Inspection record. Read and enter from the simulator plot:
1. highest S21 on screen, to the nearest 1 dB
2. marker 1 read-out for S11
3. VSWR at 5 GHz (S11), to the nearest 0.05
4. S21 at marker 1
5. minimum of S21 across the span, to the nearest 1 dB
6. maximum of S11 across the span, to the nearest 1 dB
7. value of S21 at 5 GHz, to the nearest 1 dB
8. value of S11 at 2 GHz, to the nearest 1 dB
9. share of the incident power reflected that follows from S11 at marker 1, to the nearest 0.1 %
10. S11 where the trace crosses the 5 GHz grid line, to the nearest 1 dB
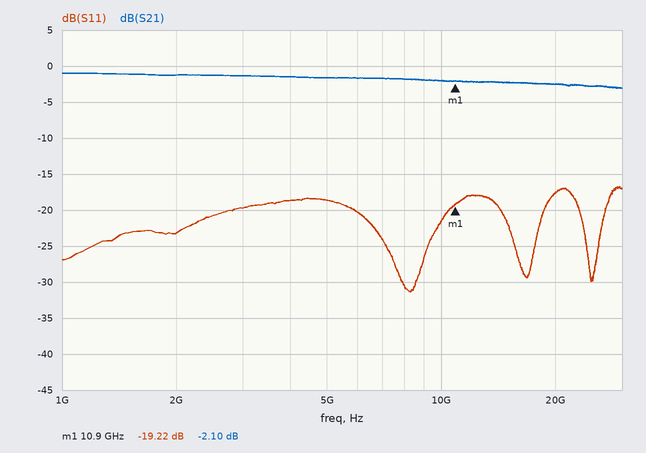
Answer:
-1 dB
-19.22 dB
1.25
-2.10 dB
-3 dB
-17 dB
-2 dB
-23 dB
1.2 %
-19 dB
